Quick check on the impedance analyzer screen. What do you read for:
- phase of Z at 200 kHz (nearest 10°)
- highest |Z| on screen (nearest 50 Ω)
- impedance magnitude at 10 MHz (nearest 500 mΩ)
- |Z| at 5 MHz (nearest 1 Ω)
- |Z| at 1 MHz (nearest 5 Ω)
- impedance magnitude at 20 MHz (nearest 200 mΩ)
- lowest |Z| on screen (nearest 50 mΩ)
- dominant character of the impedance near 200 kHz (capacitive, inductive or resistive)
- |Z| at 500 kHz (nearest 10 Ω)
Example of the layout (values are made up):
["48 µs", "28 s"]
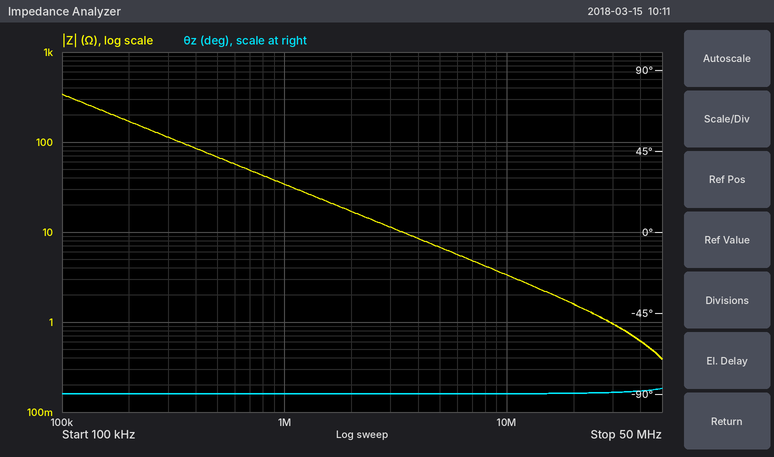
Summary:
["-90°", "350 Ω", "3.5 Ω", "7 Ω", "35 Ω", "1.6 Ω", "400 mΩ", "capacitive", "70 Ω"]
